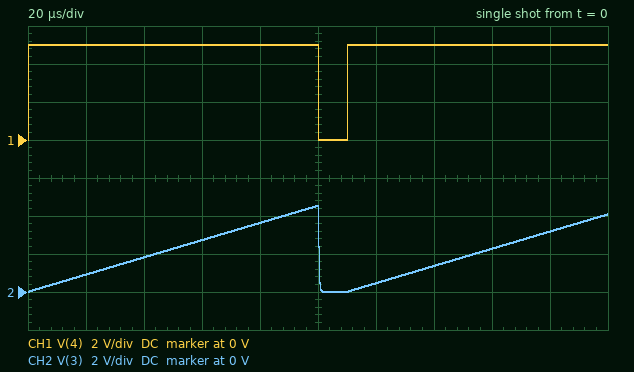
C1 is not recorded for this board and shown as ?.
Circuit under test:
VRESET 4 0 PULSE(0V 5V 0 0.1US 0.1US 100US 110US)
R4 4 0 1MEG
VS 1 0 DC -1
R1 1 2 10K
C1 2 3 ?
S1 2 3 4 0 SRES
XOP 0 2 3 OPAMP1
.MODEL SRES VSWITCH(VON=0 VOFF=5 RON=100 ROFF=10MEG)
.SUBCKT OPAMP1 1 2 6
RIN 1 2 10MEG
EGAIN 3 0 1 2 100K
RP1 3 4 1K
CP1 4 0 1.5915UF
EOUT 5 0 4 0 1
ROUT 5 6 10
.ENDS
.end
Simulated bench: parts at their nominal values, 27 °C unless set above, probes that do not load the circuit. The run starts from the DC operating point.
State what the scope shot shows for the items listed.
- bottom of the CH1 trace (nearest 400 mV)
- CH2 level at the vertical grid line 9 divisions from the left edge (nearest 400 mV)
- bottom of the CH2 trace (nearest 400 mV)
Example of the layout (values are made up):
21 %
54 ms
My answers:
0 V
3.2 V
0 V
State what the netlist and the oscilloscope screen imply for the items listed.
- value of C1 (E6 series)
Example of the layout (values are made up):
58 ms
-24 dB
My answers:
2.2 nF
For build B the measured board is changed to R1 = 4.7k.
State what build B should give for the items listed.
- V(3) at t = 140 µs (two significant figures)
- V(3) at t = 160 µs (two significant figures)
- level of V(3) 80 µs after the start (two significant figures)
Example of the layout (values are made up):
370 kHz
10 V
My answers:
2.9 V
4.8 V
7.7 V
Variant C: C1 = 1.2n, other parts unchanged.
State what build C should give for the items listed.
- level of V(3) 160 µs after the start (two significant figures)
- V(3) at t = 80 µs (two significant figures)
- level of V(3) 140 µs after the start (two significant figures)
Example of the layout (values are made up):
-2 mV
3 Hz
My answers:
4.2 V
6.6 V
2.5 V
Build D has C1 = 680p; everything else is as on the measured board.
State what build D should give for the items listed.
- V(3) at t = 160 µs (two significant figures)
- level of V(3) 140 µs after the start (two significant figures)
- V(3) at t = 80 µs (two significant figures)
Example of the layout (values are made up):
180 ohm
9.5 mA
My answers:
7.3 V
4.4 V
12 V
